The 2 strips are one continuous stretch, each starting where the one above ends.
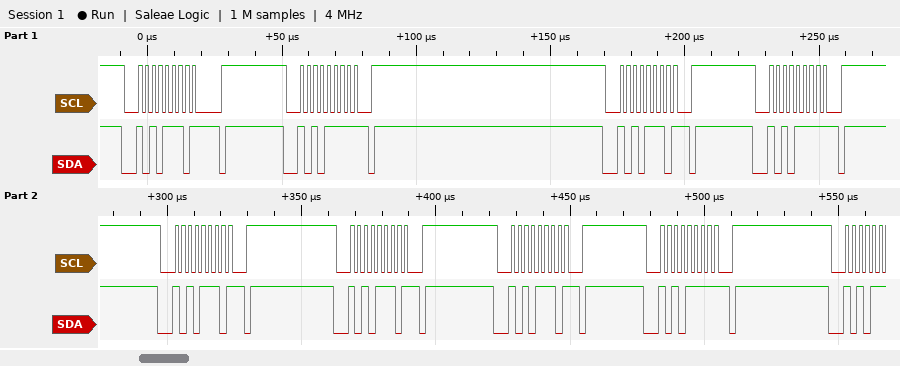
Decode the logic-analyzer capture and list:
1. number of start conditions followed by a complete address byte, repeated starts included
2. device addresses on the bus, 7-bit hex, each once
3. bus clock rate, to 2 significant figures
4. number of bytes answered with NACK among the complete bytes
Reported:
8
0x57
400 kHz
8
